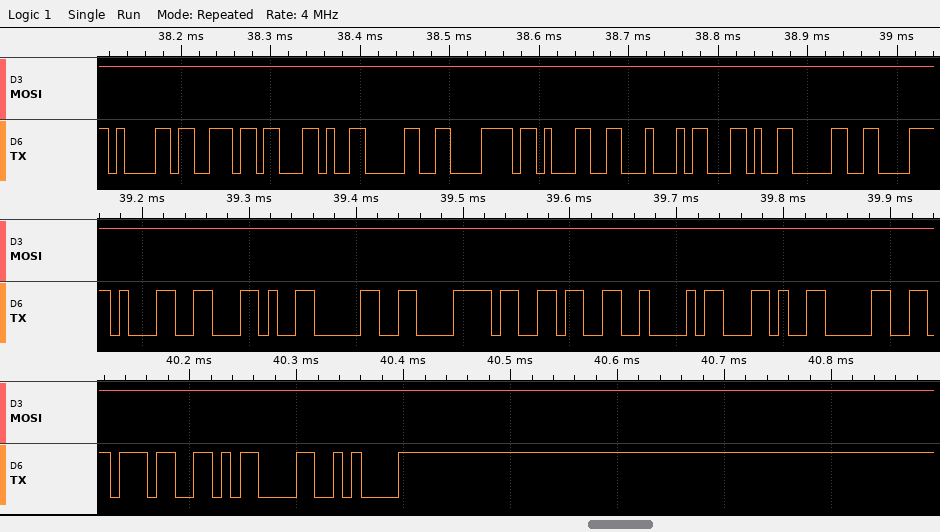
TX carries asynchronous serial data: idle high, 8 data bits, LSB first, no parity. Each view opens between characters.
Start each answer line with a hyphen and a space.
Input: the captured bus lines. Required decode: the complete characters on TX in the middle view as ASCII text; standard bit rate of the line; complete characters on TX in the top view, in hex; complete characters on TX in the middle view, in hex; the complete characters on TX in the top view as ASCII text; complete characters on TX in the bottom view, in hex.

- "1,0x6B,0"
- 115200 baud
- 61, 6E, 2C, 30, 78, 31, 44, 2C, 30
- 31, 2C, 30, 78, 36, 42, 2C, 30
- "an,0x1D,0"
- 37, 0D, 0A
